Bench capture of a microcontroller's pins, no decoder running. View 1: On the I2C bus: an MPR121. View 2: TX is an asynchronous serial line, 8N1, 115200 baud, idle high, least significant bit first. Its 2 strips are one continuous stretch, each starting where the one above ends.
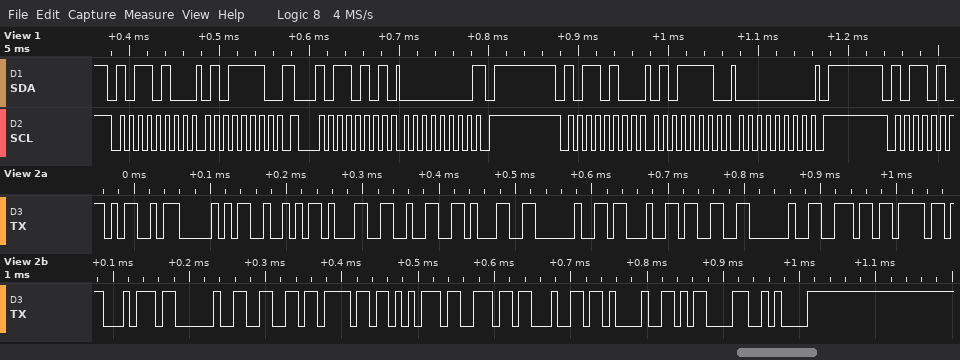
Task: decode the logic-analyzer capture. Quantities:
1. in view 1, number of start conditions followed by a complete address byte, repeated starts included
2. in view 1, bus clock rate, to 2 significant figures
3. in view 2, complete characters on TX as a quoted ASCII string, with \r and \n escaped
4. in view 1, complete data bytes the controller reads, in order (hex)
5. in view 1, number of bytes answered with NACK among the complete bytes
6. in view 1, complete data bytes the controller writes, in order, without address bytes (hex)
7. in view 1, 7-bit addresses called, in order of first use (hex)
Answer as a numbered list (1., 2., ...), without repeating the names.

1. 3
2. 100 kHz
3. "MPR121 #3 not found!\r\n"
4. 00
5. 1
6. 5E 5E 00
7. 0x5A
